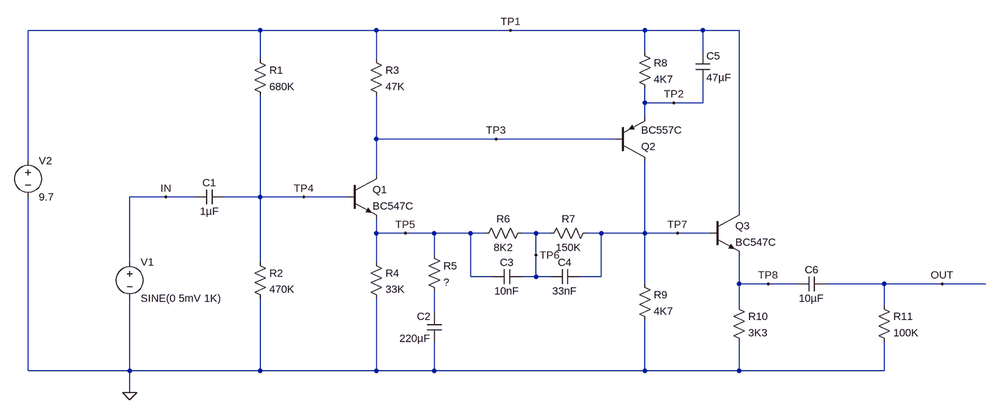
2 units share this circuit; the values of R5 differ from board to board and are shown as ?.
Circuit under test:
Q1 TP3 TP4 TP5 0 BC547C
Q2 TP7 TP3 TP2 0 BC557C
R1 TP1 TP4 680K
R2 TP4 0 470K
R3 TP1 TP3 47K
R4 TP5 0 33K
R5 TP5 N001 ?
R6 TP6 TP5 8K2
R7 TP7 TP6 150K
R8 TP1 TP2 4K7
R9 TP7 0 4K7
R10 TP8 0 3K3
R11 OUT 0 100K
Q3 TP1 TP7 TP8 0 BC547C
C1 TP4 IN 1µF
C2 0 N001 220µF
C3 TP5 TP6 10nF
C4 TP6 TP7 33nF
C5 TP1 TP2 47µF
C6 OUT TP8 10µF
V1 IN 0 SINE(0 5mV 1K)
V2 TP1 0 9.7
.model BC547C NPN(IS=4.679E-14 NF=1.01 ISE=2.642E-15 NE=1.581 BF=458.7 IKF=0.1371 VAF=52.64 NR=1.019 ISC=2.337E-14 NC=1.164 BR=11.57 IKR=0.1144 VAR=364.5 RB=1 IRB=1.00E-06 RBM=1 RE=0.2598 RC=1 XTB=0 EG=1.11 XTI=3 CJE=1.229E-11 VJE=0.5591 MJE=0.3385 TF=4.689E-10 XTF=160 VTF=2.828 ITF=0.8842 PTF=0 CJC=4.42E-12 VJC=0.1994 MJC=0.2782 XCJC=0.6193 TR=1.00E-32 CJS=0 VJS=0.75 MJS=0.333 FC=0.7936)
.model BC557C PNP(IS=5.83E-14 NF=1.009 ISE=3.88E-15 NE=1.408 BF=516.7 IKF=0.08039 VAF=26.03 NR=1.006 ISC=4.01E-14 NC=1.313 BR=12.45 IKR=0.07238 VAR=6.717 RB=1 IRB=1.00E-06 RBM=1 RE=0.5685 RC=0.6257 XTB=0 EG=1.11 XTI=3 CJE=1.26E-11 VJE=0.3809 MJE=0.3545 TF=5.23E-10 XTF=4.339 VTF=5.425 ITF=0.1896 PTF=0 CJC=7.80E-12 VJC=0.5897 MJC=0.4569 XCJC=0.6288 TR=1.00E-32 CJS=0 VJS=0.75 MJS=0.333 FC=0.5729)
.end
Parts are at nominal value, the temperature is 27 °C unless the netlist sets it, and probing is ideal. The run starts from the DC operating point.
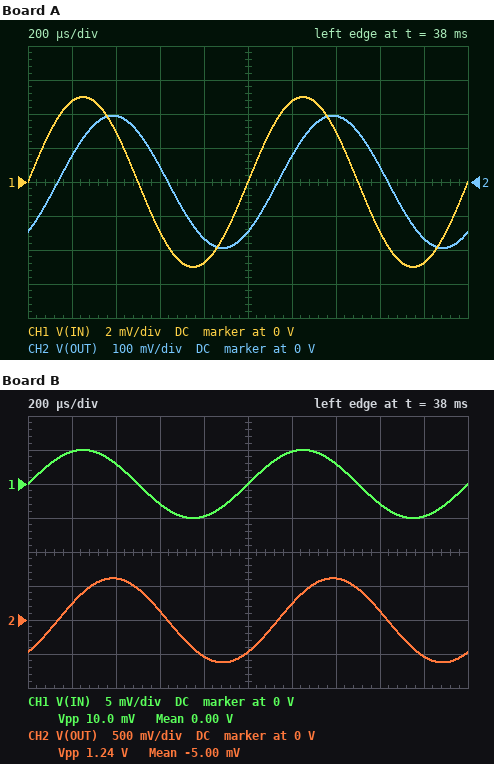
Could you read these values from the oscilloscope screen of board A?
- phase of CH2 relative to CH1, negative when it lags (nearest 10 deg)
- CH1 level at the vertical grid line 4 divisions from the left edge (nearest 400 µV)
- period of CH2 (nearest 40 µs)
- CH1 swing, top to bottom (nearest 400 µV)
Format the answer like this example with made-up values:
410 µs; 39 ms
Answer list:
-50 deg; -4.8 mV; 1.00 ms; 10.0 mV
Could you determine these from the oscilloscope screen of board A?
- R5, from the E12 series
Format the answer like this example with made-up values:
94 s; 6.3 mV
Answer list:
270 Ω
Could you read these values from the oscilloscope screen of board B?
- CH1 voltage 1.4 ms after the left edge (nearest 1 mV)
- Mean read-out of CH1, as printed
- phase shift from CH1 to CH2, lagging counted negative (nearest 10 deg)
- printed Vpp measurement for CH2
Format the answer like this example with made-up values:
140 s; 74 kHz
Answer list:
3 mV; 0.00 V; -50 deg; 1.24 V
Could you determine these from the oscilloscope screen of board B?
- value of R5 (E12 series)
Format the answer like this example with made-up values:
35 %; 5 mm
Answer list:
82 Ω
